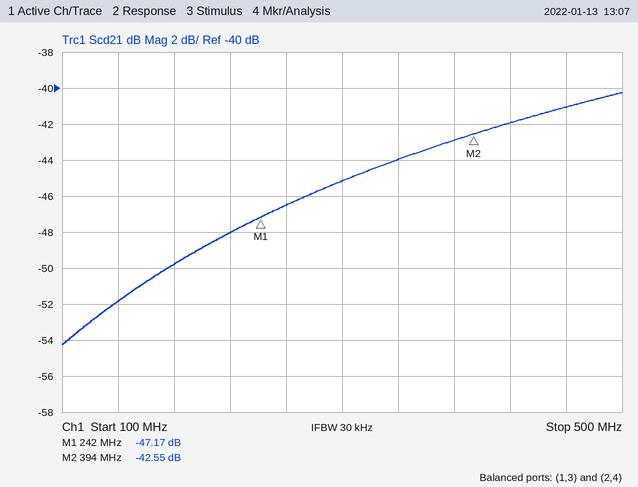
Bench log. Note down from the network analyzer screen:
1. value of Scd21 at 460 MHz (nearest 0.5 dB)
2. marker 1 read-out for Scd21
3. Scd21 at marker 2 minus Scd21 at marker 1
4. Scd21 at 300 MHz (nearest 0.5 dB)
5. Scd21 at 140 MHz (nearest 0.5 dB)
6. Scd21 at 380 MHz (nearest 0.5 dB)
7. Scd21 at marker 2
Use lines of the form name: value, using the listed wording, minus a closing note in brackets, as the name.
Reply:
value of Scd21 at 460 MHz: -41.0 dB
marker 1 read-out for Scd21: -47.17 dB
Scd21 at marker 2 minus Scd21 at marker 1: 4.62 dB
Scd21 at 300 MHz: -45.0 dB
Scd21 at 140 MHz: -52.0 dB
Scd21 at 380 MHz: -43.0 dB
Scd21 at marker 2: -42.55 dB
